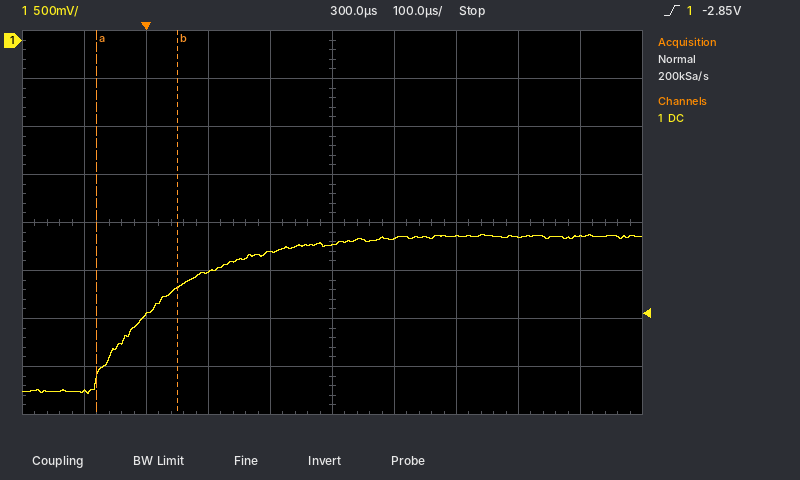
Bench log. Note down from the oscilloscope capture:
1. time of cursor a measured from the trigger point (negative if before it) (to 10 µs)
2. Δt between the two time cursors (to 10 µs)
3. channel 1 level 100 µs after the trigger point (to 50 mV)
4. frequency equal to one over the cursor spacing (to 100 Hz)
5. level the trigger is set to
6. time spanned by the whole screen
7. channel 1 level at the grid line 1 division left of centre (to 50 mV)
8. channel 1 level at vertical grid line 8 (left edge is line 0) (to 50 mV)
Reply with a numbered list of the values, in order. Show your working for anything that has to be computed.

1. -80 µs
2. 130 µs
3. -2.40 V
4. 1 / 130 µs ≈ 7.7 kHz
5. -2.85 V
6. 1 ms
7. -2.20 V
8. -2.05 V
